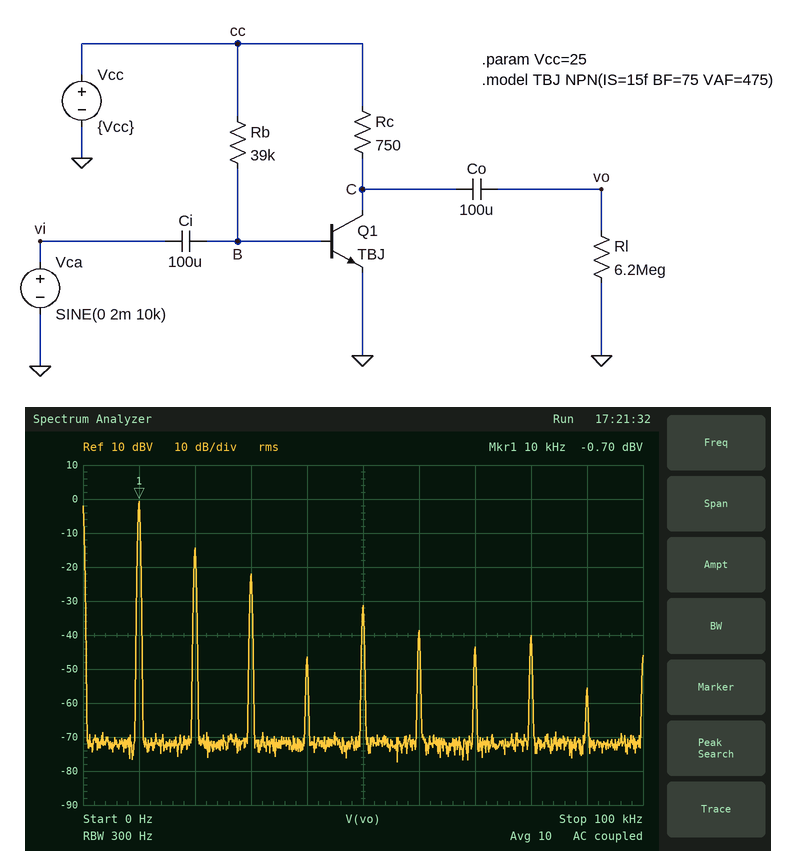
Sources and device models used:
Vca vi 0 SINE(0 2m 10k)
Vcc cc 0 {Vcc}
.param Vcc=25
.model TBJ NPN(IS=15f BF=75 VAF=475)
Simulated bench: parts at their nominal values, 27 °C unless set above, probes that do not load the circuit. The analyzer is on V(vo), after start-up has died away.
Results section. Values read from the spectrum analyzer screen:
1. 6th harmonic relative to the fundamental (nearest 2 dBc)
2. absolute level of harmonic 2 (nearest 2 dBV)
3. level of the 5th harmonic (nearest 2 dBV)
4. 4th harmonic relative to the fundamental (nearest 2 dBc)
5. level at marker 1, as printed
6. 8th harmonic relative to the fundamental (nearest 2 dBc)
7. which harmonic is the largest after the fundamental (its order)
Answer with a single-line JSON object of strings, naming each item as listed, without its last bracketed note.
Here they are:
{"6th harmonic relative to the fundamental": "-38 dBc", "absolute level of harmonic 2": "-14 dBV", "level of the 5th harmonic": "-32 dBV", "4th harmonic relative to the fundamental": "-46 dBc", "level at marker 1, as printed": "-0.70 dBV", "8th harmonic relative to the fundamental": "-40 dBc", "which harmonic is the largest after the fundamental": "2"}
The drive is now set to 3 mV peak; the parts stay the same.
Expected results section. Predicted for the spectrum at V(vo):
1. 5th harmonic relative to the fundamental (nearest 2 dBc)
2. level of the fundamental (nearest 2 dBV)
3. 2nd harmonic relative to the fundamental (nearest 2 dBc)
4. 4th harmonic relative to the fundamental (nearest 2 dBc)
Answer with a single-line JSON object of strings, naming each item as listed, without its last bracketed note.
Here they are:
{"5th harmonic relative to the fundamental": "-36 dBc", "level of the fundamental": "4 dBV", "2nd harmonic relative to the fundamental": "-16 dBc", "4th harmonic relative to the fundamental": "-34 dBc"}
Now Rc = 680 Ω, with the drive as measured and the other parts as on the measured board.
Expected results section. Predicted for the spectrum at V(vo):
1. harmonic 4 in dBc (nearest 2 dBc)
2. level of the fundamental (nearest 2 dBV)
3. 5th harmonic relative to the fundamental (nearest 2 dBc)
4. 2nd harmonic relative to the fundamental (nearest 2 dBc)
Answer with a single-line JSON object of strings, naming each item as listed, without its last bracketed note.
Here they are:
{"harmonic 4 in dBc": "-36 dBc", "level of the fundamental": "0 dBV", "5th harmonic relative to the fundamental": "-36 dBc", "2nd harmonic relative to the fundamental": "-16 dBc"}
